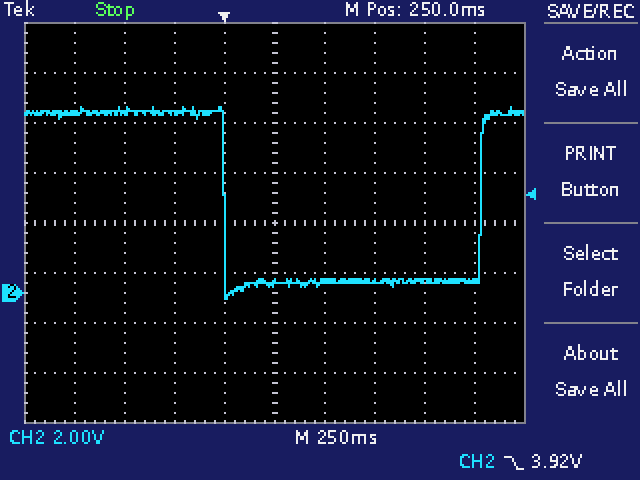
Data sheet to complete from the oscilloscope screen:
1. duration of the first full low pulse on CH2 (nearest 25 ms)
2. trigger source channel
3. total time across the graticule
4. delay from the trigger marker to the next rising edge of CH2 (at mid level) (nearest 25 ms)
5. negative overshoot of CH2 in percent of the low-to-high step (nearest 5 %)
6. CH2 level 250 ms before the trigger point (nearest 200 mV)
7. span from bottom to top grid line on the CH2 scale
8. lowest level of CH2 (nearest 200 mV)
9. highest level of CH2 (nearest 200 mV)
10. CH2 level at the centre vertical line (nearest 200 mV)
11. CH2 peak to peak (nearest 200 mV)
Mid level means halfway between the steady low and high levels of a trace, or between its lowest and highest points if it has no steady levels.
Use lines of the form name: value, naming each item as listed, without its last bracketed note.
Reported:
duration of the first full low pulse on CH2: 1.275 s
trigger source channel: CH2
total time across the graticule: 2.5 s
delay from the trigger marker to the next rising edge of CH2 (at mid level): 1.275 s
negative overshoot of CH2 in percent of the low-to-high step: 10 %
CH2 level 250 ms before the trigger point: 7.2 V
span from bottom to top grid line on the CH2 scale: 16 V
lowest level of CH2: -200 mV
highest level of CH2: 7.4 V
CH2 level at the centre vertical line: 400 mV
CH2 peak to peak: 7.6 V
